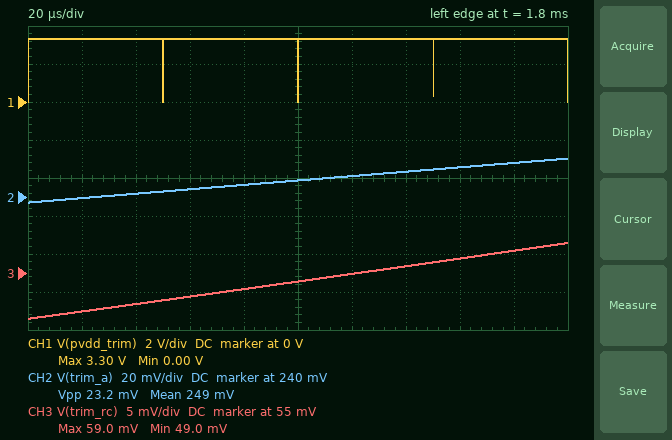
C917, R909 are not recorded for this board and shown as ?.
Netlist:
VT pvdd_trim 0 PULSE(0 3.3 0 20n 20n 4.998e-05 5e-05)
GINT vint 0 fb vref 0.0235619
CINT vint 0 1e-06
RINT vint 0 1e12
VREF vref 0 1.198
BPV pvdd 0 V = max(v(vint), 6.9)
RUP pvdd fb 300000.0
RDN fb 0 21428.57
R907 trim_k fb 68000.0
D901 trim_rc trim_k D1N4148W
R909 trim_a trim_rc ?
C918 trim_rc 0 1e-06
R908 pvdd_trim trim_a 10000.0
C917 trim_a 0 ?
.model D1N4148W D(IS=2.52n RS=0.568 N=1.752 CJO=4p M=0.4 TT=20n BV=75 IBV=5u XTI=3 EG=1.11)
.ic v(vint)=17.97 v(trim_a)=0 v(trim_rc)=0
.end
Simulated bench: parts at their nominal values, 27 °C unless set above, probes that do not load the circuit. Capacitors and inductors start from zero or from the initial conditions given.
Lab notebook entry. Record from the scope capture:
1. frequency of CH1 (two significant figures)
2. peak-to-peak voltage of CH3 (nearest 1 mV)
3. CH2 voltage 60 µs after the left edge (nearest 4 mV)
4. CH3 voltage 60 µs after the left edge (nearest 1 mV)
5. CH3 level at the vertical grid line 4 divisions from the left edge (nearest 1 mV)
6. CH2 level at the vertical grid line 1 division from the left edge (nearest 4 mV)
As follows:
20 kHz
10 mV
244 mV
52 mV
53 mV
240 mV
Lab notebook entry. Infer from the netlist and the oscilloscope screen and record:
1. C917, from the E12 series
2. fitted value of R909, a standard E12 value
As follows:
2.2 µF
3.9 kΩ
